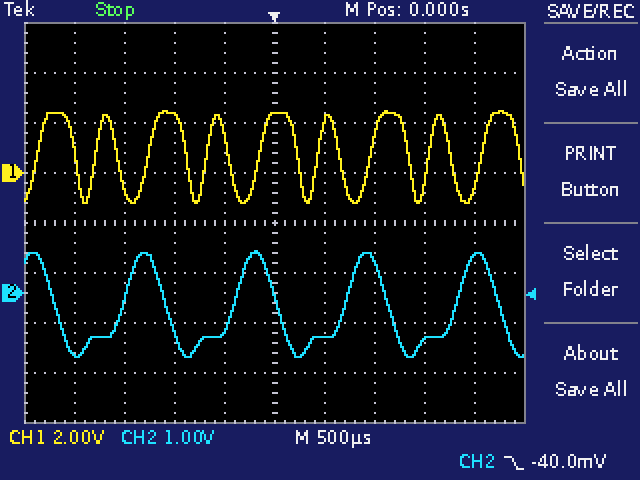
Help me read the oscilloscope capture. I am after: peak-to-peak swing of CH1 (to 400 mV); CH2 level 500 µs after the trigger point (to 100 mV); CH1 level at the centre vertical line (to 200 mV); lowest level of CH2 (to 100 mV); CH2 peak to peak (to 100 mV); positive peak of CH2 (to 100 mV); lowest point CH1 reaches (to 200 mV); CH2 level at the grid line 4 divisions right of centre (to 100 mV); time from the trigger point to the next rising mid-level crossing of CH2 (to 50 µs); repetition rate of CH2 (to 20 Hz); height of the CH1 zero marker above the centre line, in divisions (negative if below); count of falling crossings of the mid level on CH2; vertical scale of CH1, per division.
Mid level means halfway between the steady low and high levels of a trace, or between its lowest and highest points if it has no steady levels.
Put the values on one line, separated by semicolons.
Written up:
3.6 V; -900 mV; 2.4 V; -1.3 V; 2.1 V; 800 mV; -1.2 V; 700 mV; 700 µs; 900 Hz; +1.0 div; 5; 2 V
